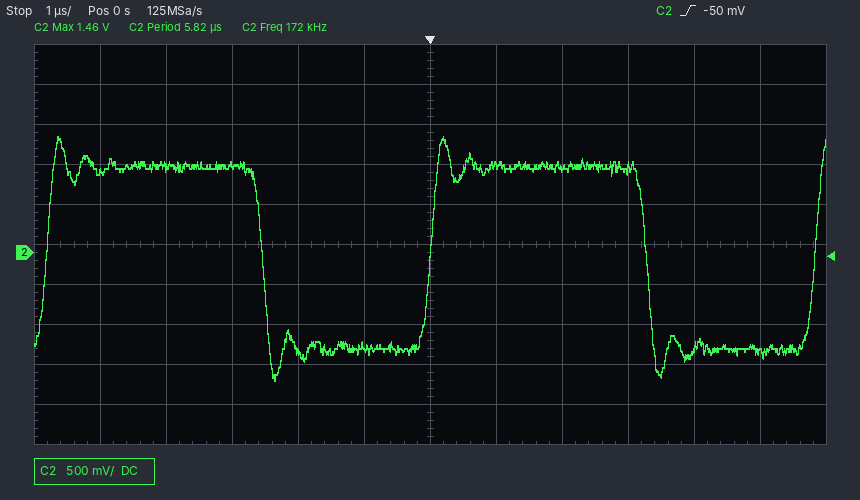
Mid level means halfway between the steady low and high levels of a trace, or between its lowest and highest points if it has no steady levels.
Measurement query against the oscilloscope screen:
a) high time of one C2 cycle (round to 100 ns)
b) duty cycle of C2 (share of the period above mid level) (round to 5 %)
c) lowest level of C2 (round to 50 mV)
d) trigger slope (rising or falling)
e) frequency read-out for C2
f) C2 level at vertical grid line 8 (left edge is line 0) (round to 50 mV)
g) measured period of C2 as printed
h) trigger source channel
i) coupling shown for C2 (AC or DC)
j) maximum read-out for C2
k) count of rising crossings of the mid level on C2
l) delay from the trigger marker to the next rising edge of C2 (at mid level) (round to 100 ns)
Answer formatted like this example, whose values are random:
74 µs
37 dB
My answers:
3.3 µs
55 %
-1.60 V
rising
172 kHz
1.05 V
5.82 µs
C2
DC
1.46 V
3
5.8 µs
